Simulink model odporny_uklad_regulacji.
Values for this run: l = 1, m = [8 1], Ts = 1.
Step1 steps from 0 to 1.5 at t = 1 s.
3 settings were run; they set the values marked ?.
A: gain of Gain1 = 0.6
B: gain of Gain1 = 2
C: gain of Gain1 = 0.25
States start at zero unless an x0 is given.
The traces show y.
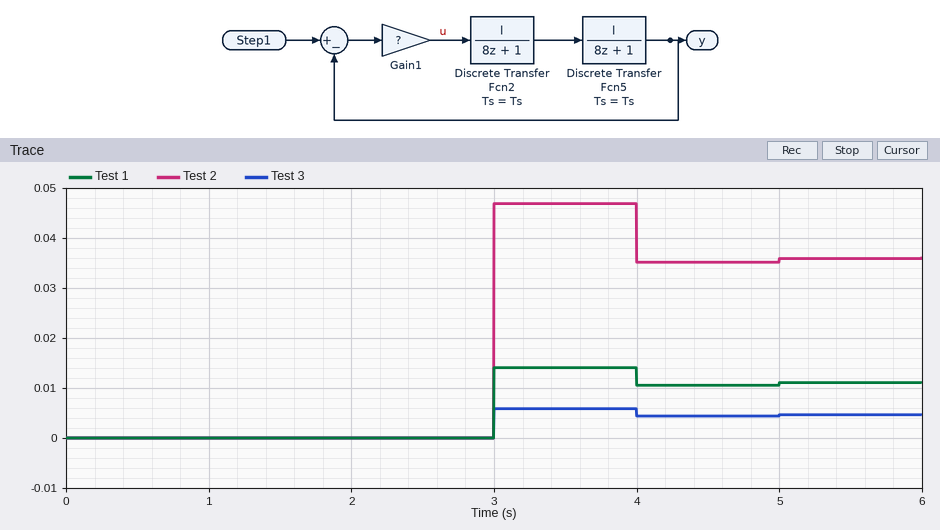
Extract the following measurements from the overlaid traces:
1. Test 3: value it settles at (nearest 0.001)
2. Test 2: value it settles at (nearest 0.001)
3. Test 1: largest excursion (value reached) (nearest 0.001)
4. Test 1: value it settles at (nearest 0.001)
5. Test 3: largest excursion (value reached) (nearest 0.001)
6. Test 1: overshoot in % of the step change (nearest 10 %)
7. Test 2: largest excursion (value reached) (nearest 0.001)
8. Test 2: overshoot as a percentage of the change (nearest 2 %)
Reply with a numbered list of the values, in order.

1. 0.005
2. 0.036
3. 0.014
4. 0.011
5. 0.006
6. 30 %
7. 0.047
8. 30 %
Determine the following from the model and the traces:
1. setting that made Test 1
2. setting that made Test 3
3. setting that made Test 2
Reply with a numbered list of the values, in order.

1. A
2. C
3. B
